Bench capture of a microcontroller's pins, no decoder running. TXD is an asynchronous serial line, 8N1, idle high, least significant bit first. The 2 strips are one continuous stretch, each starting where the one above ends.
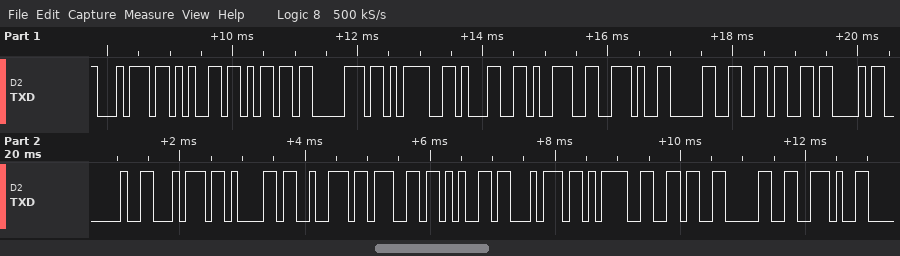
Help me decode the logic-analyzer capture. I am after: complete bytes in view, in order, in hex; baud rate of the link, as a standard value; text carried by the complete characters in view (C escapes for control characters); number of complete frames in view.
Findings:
74 65 6D 70 3D 31 39 2E 30 36 43 20 74 61 72 67 65 74 3D 36 30 2E
9600 baud
"temp=19.06C target=60."
22
